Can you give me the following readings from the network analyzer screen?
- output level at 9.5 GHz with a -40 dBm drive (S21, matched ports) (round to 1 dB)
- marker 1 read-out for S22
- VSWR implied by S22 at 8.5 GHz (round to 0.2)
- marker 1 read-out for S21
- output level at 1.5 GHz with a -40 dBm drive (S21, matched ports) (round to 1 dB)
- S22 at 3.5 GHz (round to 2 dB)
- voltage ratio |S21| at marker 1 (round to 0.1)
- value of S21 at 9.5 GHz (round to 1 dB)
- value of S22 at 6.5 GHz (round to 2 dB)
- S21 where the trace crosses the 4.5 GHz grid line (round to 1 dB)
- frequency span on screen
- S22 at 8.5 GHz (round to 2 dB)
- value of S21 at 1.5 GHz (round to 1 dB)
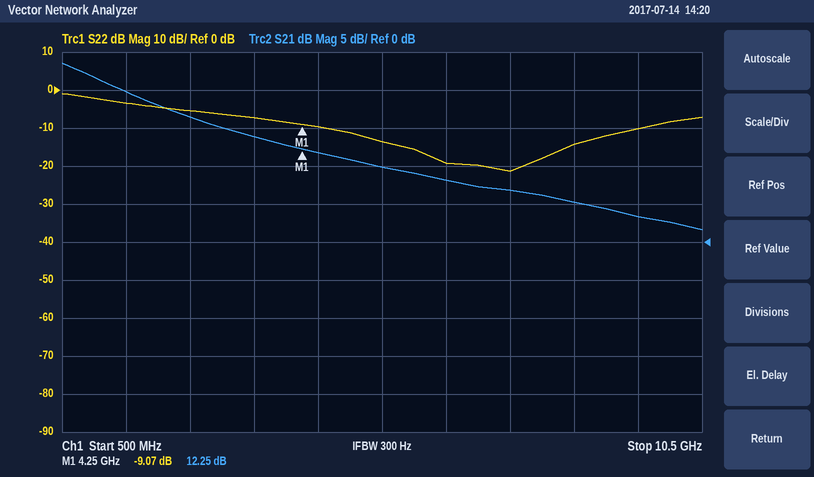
-37 dBm
-9.07 dB
1.4
12.25 dB
-20 dBm
-8 dB
4.1
3 dB
-20 dB
12 dB
10 GHz
-14 dB
20 dB
